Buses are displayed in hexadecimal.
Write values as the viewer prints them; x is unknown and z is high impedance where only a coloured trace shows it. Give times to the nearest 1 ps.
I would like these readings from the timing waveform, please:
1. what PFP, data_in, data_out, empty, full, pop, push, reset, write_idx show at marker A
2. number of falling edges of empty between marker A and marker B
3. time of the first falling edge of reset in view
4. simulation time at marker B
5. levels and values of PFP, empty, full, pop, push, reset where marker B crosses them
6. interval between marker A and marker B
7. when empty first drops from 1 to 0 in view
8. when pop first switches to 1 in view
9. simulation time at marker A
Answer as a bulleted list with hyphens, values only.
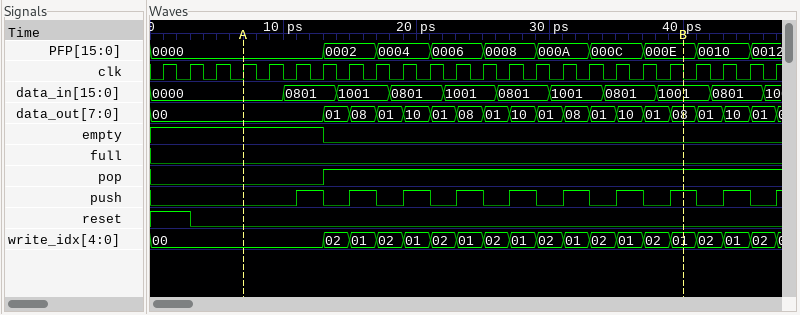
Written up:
- PFP=0000, data_in=0000, data_out=00, empty=1, full=0, pop=0, push=0, reset=0, write_idx=00
- 1
- 3 ps
- 40 ps
- PFP=000E, empty=0, full=0, pop=1, push=1, reset=0
- 33 ps
- 13 ps
- 13 ps
- 7 ps
